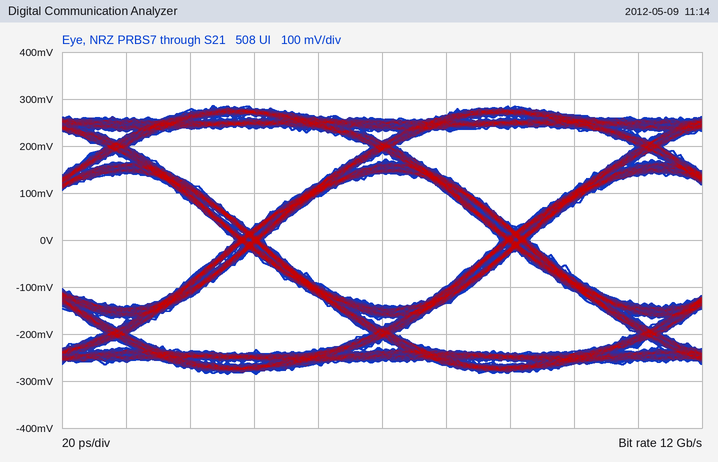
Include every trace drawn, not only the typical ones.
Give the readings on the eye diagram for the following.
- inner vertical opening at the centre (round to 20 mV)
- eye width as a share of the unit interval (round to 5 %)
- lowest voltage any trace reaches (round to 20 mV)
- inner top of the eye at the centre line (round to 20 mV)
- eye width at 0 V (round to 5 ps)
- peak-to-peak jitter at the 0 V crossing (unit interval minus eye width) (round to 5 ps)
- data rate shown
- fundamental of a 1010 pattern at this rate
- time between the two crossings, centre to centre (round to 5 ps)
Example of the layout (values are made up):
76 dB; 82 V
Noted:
280 mV; 90 %; -280 mV; 140 mV; 75 ps; 10 ps; 12 Gb/s; 6 GHz; 85 ps
